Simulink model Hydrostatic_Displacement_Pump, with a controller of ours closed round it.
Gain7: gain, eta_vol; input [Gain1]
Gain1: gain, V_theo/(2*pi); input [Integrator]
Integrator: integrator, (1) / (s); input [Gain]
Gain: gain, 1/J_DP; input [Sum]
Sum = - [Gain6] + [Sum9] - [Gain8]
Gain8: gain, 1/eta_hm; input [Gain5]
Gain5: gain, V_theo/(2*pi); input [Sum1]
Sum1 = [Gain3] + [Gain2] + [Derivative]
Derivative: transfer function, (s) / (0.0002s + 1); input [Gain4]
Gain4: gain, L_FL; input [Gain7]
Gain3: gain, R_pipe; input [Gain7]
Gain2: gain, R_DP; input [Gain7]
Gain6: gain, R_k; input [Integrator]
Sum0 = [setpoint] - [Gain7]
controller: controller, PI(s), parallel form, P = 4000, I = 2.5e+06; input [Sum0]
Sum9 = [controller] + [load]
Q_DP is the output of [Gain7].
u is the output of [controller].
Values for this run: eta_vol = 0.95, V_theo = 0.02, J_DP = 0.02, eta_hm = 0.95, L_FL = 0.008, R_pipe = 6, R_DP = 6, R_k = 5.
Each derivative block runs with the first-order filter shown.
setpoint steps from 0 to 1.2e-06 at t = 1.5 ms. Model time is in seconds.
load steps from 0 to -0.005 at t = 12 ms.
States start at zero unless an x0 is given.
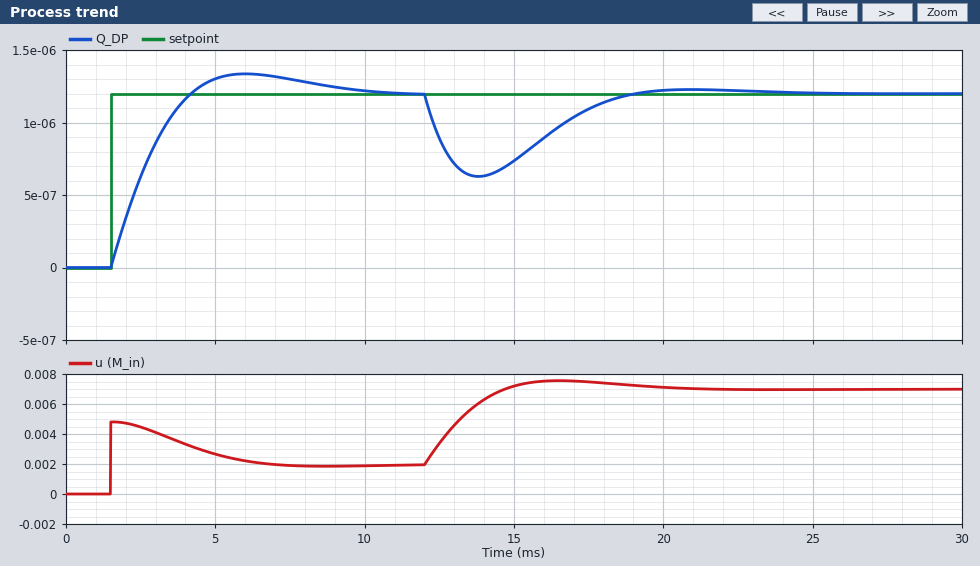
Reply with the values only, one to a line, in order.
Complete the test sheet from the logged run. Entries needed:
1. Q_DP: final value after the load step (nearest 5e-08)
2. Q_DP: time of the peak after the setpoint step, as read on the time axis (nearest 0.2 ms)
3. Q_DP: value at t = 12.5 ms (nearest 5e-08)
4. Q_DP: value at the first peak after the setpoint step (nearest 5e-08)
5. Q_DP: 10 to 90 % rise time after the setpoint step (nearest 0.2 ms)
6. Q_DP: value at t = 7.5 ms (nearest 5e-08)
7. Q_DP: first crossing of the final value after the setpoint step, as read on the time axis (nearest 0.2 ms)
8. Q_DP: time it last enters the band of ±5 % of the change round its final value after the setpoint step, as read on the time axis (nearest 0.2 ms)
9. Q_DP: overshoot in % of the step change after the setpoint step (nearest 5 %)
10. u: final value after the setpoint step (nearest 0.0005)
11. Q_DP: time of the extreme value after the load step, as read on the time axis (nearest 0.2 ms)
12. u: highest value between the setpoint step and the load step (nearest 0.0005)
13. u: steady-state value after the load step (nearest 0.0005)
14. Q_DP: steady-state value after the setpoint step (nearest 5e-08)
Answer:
0.00000120
6.0 ms
0.00000090
0.00000135
2.0 ms
0.00000130
4.2 ms
8.6 ms
10 %
0.0020
13.8 ms
0.0050
0.0070
0.00000120
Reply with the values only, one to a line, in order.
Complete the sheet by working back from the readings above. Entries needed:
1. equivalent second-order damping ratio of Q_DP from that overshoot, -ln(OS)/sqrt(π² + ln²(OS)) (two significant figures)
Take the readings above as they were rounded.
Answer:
0.59
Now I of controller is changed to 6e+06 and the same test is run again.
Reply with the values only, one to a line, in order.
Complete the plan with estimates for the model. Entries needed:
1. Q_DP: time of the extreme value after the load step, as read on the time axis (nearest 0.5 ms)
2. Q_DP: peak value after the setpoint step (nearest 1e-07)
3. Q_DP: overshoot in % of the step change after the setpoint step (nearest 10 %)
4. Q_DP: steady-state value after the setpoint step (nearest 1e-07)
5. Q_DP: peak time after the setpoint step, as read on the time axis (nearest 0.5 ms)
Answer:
13.5 ms
0.0000015
30 %
0.0000012
4.5 ms
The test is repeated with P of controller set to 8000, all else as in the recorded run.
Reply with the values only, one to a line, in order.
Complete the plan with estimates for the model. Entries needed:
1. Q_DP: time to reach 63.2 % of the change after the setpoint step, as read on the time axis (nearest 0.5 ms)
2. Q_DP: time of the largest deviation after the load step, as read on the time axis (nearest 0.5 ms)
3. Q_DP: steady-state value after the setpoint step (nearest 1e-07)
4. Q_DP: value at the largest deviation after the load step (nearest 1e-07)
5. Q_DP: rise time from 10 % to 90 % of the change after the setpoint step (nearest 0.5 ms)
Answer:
2.5 ms
13.5 ms
0.0000012
0.0000008
1.5 ms
